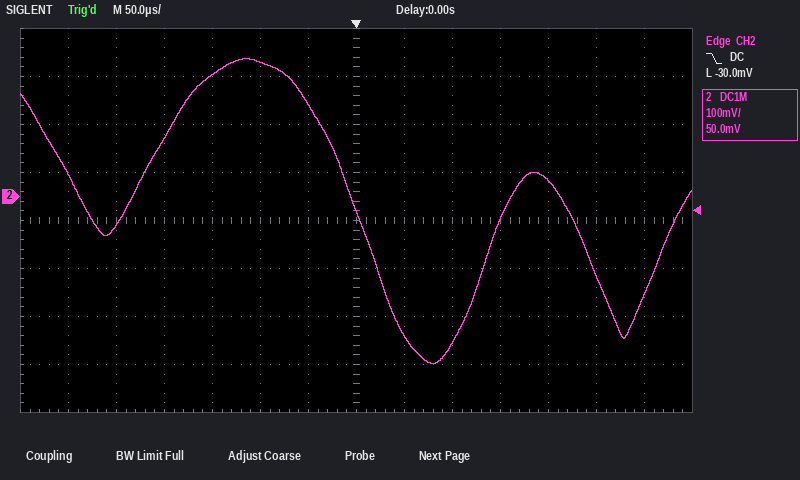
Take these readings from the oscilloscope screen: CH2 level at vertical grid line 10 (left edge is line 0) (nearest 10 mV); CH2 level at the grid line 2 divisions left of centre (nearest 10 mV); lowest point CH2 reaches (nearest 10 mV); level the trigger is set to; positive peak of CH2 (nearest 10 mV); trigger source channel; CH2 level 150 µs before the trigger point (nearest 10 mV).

-50 mV
280 mV
-350 mV
-30.0 mV
290 mV
CH2
250 mV
